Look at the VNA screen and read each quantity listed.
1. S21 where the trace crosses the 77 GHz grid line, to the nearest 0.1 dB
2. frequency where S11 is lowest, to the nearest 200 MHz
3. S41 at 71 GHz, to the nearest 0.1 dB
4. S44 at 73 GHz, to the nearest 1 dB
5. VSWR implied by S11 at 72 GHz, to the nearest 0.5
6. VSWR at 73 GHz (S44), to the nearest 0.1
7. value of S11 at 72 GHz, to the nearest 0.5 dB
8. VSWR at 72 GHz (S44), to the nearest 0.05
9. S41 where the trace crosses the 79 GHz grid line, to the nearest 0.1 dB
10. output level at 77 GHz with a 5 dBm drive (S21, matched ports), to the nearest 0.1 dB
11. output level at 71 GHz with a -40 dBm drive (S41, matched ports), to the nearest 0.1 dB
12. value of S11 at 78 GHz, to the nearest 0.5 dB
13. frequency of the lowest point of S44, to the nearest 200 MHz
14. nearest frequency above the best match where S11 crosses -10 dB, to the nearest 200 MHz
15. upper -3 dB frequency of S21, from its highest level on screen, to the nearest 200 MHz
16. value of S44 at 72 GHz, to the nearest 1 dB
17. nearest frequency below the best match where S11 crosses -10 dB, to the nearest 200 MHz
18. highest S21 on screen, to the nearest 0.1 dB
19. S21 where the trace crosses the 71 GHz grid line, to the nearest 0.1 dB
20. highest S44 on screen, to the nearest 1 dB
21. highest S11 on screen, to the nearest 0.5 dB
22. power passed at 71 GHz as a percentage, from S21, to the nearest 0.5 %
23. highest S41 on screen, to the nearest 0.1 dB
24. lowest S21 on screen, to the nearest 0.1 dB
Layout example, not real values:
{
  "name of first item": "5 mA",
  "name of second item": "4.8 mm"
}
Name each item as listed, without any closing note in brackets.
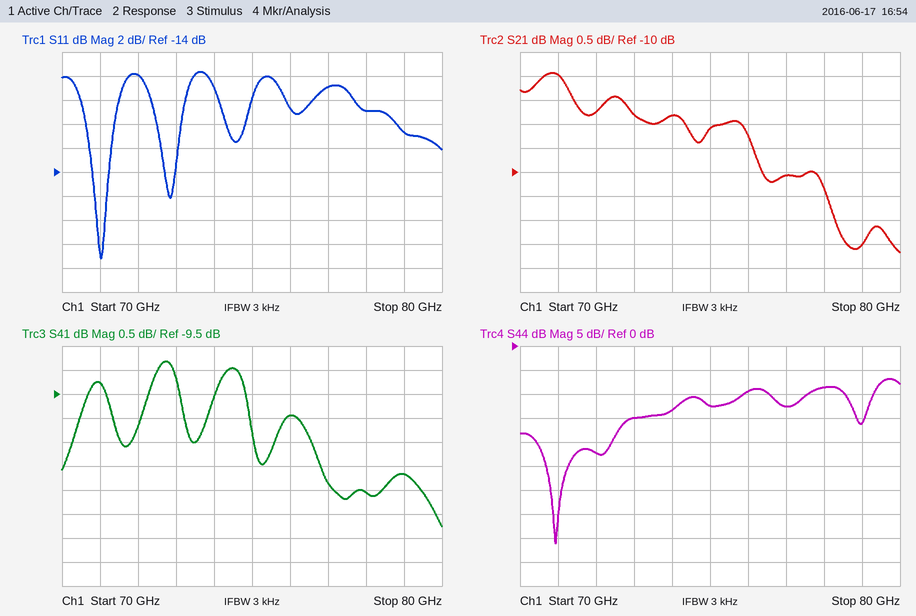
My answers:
{
  "S21 where the trace crosses the 77 GHz grid line, to the nearest 0.1 dB": "-10.1 dB",
  "frequency where S11 is lowest, to the nearest 200 MHz": "71.0 GHz",
  "S41 at 71 GHz, to the nearest 0.1 dB": "-9.3 dB",
  "S44 at 73 GHz, to the nearest 1 dB": "-15 dB",
  "VSWR implied by S11 at 72 GHz, to the nearest 0.5": "3.0",
  "VSWR at 73 GHz (S44), to the nearest 0.1": "1.4",
  "value of S11 at 72 GHz, to the nearest 0.5 dB": "-6.0 dB",
  "VSWR at 72 GHz (S44), to the nearest 0.05": "1.15",
  "S41 where the trace crosses the 79 GHz grid line, to the nearest 0.1 dB": "-11.2 dB",
  "output level at 77 GHz with a 5 dBm drive (S21, matched ports), to the nearest 0.1 dB": "-5.1 dBm",
  "output level at 71 GHz with a -40 dBm drive (S41, matched ports), to the nearest 0.1 dB": "-49.3 dBm",
  "value of S11 at 78 GHz, to the nearest 0.5 dB": "-9.0 dB",
  "frequency of the lowest point of S44, to the nearest 200 MHz": "71.0 GHz",
  "nearest frequency above the best match where S11 crosses -10 dB, to the nearest 200 MHz": "71.4 GHz",
  "upper -3 dB frequency of S21, from its highest level on screen, to the nearest 200 MHz": "78.2 GHz",
  "value of S44 at 72 GHz, to the nearest 1 dB": "-22 dB",
  "nearest frequency below the best match where S11 crosses -10 dB, to the nearest 200 MHz": "70.6 GHz",
  "highest S21 on screen, to the nearest 0.1 dB": "-7.9 dB",
  "S21 where the trace crosses the 71 GHz grid line, to the nearest 0.1 dB": "-8.0 dB",
  "highest S44 on screen, to the nearest 1 dB": "-7 dB",
  "highest S11 on screen, to the nearest 0.5 dB": "-5.5 dB",
  "power passed at 71 GHz as a percentage, from S21, to the nearest 0.5 %": "16.0 %",
  "highest S41 on screen, to the nearest 0.1 dB": "-8.8 dB",
  "lowest S21 on screen, to the nearest 0.1 dB": "-11.7 dB"
}
